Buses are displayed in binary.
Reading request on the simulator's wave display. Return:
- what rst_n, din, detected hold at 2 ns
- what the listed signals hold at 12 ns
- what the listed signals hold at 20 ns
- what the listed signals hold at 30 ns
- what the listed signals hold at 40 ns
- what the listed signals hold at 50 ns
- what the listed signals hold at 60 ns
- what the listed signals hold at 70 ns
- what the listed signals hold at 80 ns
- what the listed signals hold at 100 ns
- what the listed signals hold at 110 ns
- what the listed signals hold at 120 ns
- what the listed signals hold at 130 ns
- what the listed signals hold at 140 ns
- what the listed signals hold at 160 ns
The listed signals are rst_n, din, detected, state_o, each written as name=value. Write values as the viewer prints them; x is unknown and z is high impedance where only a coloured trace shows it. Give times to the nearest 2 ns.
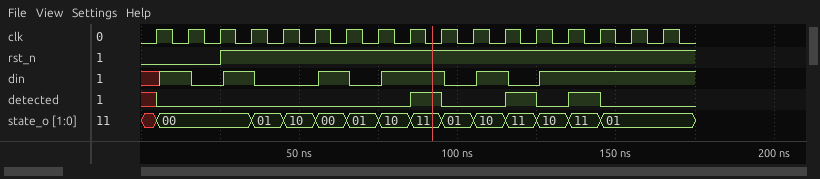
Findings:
rst_n=0, din=x, detected=x
rst_n=0, din=1, detected=0, state_o=00
rst_n=0, din=0, detected=0, state_o=00
rst_n=1, din=1, detected=0, state_o=00
rst_n=1, din=0, detected=0, state_o=01
rst_n=1, din=0, detected=0, state_o=10
rst_n=1, din=1, detected=0, state_o=00
rst_n=1, din=0, detected=0, state_o=01
rst_n=1, din=1, detected=0, state_o=10
rst_n=1, din=0, detected=0, state_o=01
rst_n=1, din=1, detected=0, state_o=10
rst_n=1, din=0, detected=1, state_o=11
rst_n=1, din=1, detected=0, state_o=10
rst_n=1, din=1, detected=1, state_o=11
rst_n=1, din=1, detected=0, state_o=01
